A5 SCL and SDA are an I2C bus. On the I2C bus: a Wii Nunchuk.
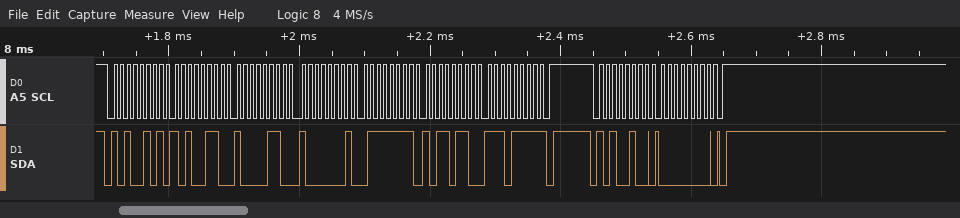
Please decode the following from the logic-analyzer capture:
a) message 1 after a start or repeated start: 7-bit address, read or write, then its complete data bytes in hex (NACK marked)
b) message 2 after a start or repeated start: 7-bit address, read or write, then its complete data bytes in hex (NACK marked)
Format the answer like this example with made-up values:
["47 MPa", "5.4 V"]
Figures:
["0x52 read: A6 86 81 7F B6 EF NACK", "0x52 write: 00"]
